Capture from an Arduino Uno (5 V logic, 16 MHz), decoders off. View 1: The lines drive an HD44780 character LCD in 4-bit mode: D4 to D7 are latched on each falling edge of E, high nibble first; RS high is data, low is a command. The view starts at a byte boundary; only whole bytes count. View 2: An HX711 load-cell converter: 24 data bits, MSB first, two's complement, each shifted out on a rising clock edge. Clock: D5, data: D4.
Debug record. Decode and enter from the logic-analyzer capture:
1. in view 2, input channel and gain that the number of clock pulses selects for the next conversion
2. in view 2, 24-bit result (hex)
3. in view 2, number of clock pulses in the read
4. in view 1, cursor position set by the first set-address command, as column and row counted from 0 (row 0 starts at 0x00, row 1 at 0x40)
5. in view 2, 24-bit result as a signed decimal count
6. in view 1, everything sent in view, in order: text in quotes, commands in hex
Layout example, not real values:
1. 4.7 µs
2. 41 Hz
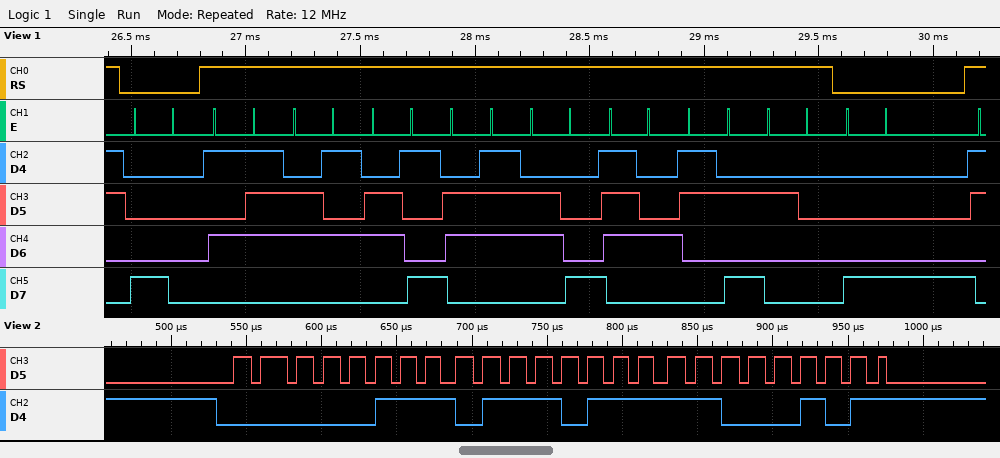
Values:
1. channel A, gain 128
2. 0x0777C5
3. 25
4. column 0, row 0
5. 489413
6. 0x80 "Weight: " 0x88
